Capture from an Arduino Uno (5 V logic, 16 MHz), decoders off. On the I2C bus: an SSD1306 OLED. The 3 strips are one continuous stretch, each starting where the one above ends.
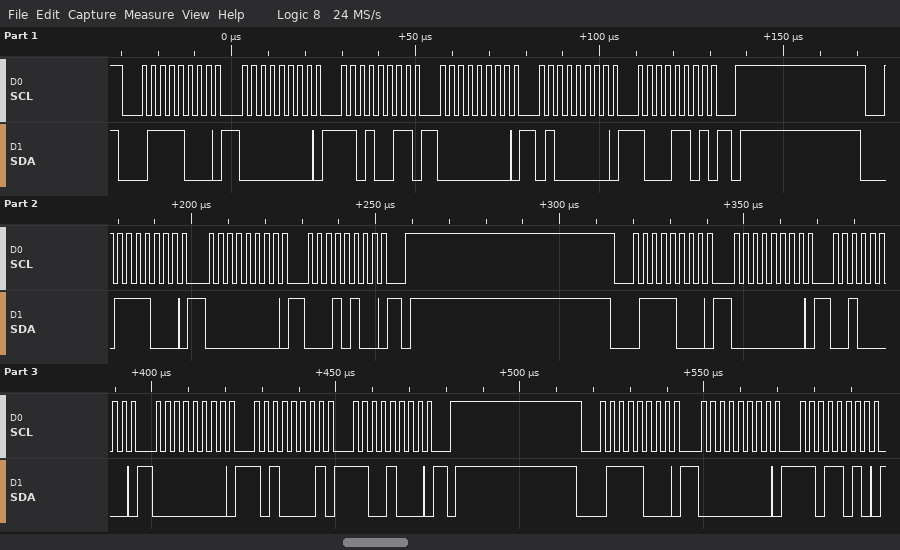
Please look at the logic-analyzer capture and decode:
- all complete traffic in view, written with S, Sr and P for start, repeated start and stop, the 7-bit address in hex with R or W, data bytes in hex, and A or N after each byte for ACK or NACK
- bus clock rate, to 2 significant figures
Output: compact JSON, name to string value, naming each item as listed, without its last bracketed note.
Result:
{"all complete traffic in view, written with S, Sr and P for start, repeated start and stop, the 7-bit address in hex with R or W, data bytes in hex, and A or N after each byte for ACK or NACK": "S 3CW A 00 A D3 A 00 A 40 A 8D A P S 3CW A 00 A 14 A P S 3CW A 00 A 20 A 00 A A1 A C8 A P S 3CW A 00 A DA A", "bus clock rate, to 2 significant figures": "400 kHz"}
